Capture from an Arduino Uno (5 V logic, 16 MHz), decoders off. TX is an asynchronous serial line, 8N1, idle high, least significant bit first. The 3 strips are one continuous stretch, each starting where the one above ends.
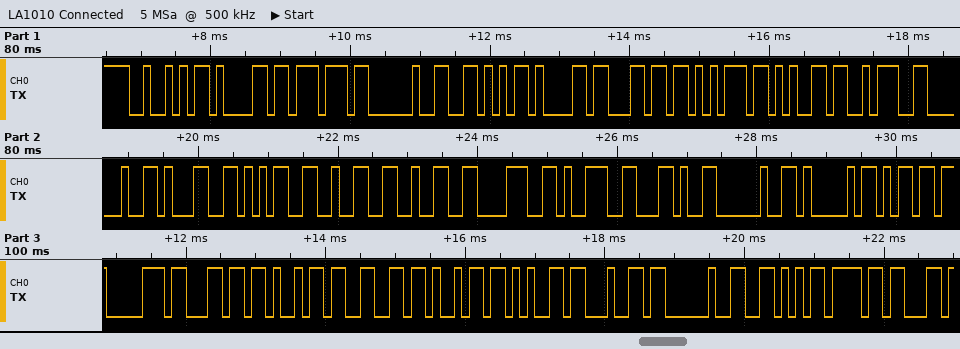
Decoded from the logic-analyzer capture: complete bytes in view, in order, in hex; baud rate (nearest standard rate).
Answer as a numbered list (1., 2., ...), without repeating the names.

1. 52 61 77 20 56 61 6C 75 65 3A 20 31 35 32 32 38 39 2C 20 41 6D 70 6C 69 66 69 65 64 20 56 6F
2. 9600 baud
